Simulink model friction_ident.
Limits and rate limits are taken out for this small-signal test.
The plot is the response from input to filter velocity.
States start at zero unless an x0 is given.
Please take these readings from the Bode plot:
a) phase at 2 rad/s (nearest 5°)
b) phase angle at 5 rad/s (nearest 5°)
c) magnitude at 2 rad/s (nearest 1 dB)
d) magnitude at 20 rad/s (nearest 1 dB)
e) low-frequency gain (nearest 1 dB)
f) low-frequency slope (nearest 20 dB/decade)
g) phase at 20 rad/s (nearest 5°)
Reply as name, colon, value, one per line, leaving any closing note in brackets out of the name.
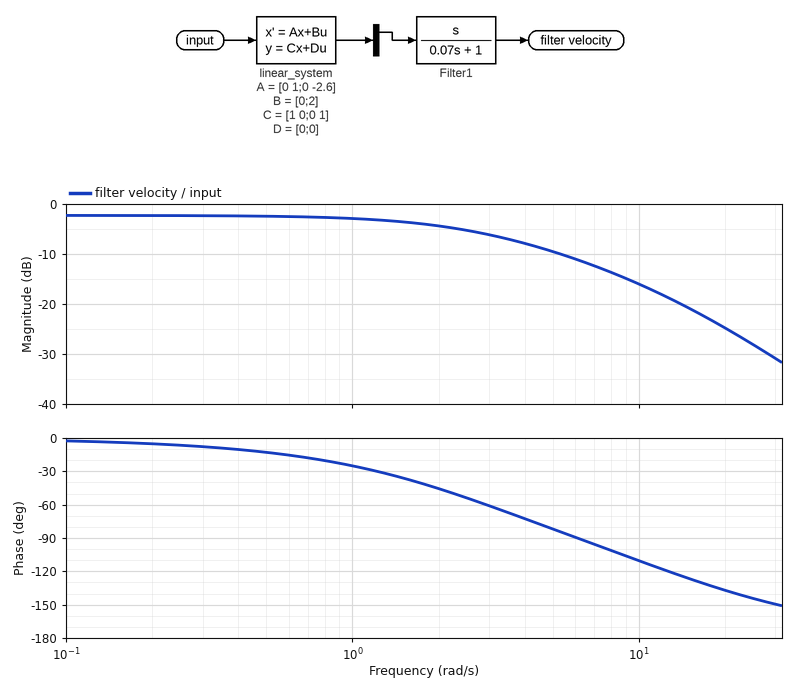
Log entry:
phase at 2 rad/s: -45°
phase angle at 5 rad/s: -80°
magnitude at 2 rad/s: -4 dB
magnitude at 20 rad/s: -25 dB
low-frequency gain: -2 dB
low-frequency slope: 0 dB/decade
phase at 20 rad/s: -135°
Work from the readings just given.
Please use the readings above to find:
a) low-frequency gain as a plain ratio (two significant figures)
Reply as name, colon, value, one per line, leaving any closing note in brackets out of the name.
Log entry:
low-frequency gain as a plain ratio: 0.79
